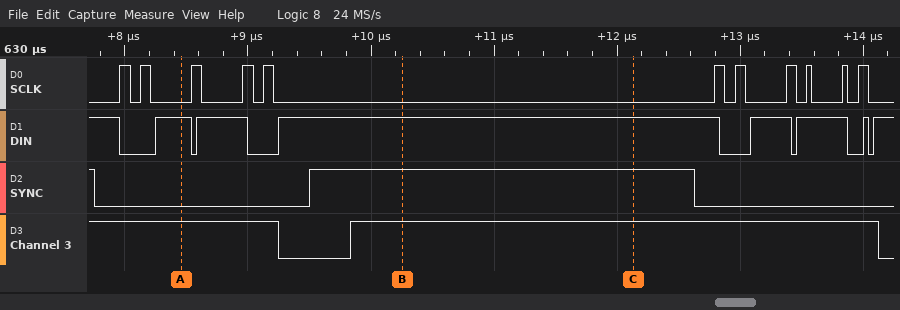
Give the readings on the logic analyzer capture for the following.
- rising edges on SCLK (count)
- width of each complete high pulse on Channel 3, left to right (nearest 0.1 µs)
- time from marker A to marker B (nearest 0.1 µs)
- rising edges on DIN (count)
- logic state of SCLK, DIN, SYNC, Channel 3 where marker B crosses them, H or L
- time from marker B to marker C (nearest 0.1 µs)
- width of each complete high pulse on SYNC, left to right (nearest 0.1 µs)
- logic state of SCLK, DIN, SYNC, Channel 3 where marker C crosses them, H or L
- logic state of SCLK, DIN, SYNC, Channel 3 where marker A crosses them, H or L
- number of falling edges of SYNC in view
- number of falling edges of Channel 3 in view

11
4.3 µs
1.8 µs
7
SCLK=L, DIN=H, SYNC=H, Channel 3=H
1.9 µs
3.1 µs
SCLK=L, DIN=H, SYNC=H, Channel 3=H
SCLK=L, DIN=H, SYNC=L, Channel 3=H
2
2
